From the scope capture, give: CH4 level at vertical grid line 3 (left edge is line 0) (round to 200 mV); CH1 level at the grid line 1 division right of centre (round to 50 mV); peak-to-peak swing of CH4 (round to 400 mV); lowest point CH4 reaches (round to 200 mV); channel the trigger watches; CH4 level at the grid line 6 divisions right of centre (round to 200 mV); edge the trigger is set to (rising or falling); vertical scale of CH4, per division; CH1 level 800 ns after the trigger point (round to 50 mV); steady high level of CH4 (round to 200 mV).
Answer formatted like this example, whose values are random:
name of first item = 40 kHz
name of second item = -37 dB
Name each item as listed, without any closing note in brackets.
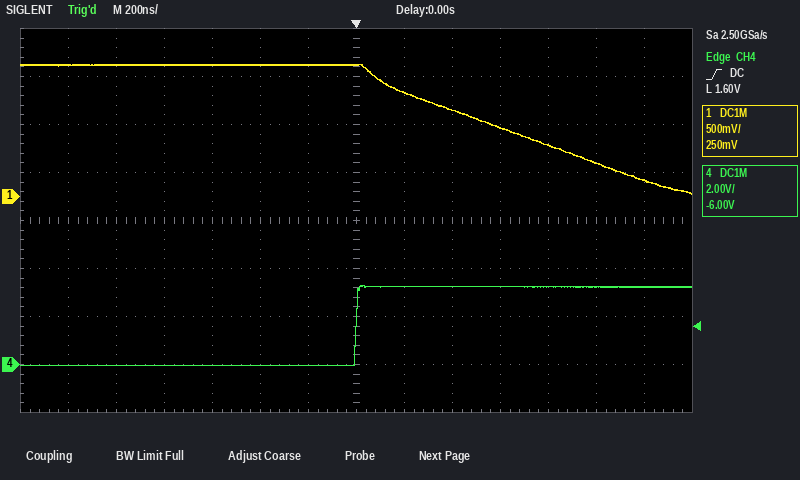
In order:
CH4 level at vertical grid line 3 (left edge is line 0) = 0.0 V
CH1 level at the grid line 1 division right of centre = 1.10 V
peak-to-peak swing of CH4 = 3.2 V
lowest point CH4 reaches = 0.0 V
channel the trigger watches = CH4
CH4 level at the grid line 6 divisions right of centre = 3.2 V
edge the trigger is set to = rising
vertical scale of CH4, per division = 2 V
CH1 level 800 ns after the trigger point = 550 mV
steady high level of CH4 = 3.2 V
